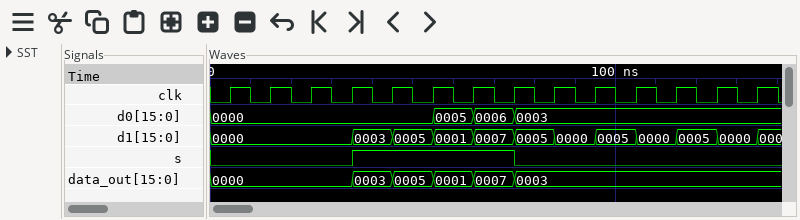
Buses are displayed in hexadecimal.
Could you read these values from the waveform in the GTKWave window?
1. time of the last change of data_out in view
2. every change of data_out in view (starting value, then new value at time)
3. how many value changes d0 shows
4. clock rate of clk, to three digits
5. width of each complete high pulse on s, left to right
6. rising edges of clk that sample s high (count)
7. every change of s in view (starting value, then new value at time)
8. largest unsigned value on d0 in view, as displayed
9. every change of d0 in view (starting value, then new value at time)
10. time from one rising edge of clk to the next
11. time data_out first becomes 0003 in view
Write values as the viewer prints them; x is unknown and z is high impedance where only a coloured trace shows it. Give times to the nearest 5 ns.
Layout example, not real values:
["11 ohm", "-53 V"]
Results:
["75 ns", "0000, 0003 at 35 ns, 0005 at 45 ns, 0001 at 55 ns, 0007 at 65 ns, 0003 at 75 ns", "3", "100 MHz", "40 ns", "4", "0, 1 at 35 ns, 0 at 75 ns", "0006", "0000, 0005 at 55 ns, 0006 at 65 ns, 0003 at 75 ns", "10 ns", "35 ns"]
